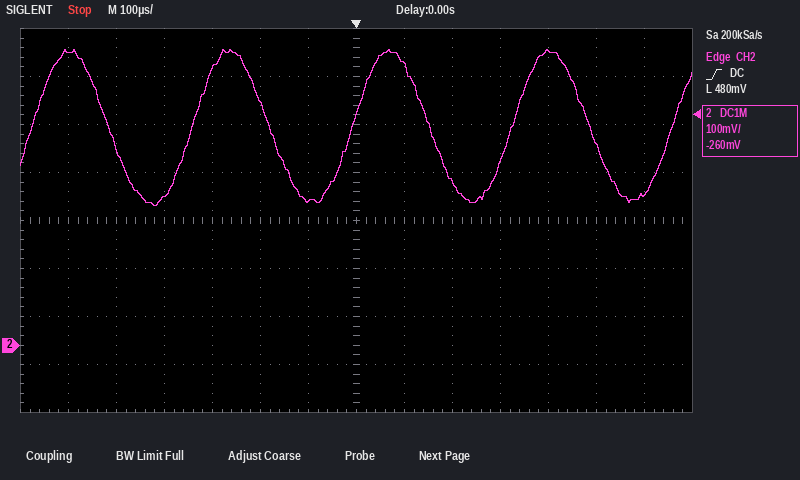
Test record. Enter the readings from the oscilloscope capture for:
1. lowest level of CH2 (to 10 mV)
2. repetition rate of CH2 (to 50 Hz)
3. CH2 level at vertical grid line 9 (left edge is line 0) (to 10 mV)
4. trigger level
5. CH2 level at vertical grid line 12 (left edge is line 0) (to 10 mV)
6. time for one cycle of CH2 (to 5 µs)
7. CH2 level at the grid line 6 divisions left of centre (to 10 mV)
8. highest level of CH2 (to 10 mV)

290 mV
3.00 kHz
340 mV
480 mV
420 mV
335 µs
610 mV
620 mV
